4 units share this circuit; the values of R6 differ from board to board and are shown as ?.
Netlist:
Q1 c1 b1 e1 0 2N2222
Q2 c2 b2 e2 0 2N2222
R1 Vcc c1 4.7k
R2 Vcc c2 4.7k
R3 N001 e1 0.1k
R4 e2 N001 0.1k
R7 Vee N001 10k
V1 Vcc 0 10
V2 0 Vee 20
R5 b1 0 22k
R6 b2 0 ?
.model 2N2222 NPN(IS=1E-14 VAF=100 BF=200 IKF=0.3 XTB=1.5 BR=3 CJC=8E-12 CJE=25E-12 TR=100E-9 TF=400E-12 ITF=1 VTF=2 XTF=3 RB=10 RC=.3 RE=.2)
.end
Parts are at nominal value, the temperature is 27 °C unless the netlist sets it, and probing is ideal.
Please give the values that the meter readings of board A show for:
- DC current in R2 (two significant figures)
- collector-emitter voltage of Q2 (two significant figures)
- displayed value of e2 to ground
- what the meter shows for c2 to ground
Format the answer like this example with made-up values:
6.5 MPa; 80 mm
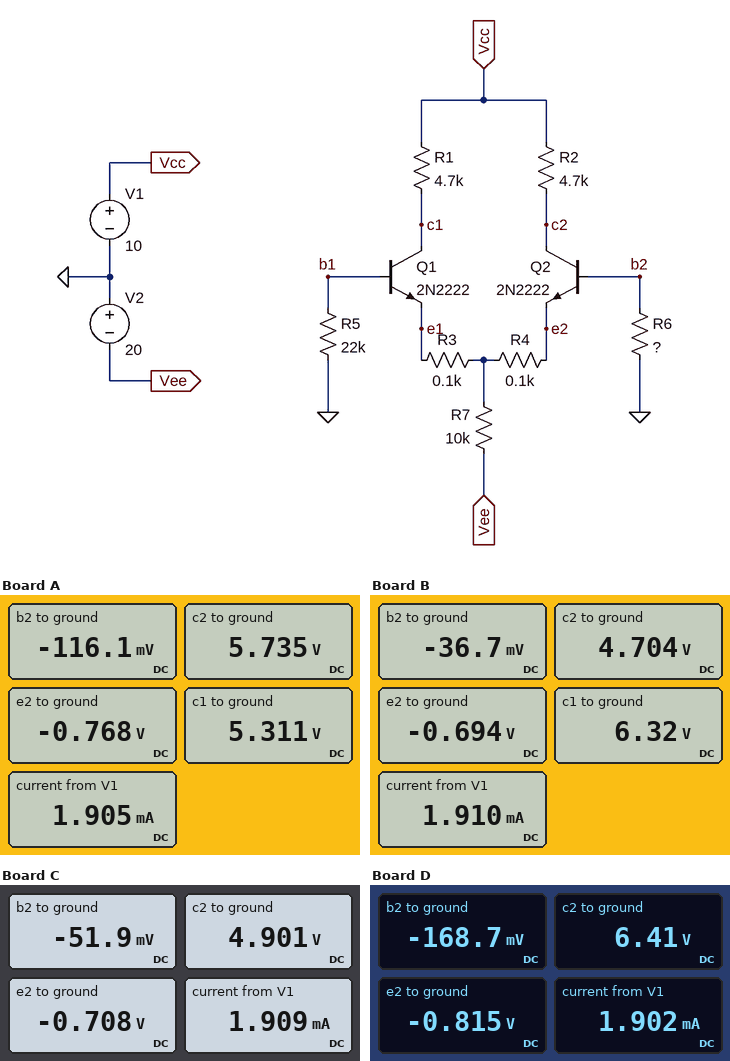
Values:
910 µA; 6.5 V; -0.768 V; 5.735 V
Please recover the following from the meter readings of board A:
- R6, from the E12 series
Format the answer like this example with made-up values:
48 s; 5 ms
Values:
27 kΩ
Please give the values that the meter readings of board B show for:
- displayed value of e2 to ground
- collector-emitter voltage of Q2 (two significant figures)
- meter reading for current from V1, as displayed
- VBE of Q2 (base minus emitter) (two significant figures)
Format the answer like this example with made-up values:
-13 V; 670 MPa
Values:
-0.694 V; 5.4 V; 1.910 mA; 660 mV
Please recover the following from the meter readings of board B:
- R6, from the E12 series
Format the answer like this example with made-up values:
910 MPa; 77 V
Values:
6.8 kΩ
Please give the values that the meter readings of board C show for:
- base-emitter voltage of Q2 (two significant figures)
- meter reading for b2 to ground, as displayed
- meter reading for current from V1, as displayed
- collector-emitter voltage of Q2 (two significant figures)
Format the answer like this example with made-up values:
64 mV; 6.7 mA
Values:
660 mV; -51.9 mV; 1.909 mA; 5.6 V
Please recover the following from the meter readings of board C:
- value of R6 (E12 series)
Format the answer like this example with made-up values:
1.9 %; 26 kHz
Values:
10 kΩ
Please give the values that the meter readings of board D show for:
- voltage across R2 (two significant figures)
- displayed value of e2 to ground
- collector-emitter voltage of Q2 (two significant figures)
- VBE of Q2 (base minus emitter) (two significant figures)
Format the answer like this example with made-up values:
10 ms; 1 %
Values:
3.6 V; -0.815 V; 7.2 V; 650 mV
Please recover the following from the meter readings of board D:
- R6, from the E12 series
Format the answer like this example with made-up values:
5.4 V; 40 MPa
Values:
47 kΩ
